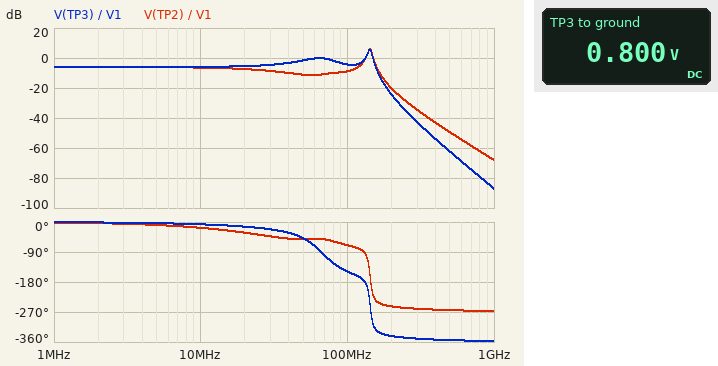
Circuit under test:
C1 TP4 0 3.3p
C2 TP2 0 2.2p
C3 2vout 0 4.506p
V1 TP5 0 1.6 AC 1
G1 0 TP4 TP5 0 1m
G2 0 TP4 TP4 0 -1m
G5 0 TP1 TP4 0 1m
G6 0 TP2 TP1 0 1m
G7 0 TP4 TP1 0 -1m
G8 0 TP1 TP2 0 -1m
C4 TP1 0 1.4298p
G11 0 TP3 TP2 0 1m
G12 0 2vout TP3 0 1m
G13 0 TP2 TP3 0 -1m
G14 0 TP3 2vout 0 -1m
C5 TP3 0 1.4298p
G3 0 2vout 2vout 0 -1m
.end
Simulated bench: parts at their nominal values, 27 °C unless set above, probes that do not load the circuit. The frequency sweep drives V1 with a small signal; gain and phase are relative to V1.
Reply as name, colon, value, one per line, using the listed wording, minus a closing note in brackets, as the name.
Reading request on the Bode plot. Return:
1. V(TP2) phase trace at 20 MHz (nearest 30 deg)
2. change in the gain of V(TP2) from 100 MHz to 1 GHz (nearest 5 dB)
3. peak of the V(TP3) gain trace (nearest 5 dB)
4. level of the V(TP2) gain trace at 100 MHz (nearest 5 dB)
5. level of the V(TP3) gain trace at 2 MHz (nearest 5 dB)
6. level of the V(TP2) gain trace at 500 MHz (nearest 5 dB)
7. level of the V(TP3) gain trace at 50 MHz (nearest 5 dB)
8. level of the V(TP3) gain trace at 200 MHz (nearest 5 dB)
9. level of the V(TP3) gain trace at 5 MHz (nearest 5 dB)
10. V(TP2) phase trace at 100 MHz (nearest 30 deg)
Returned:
V(TP2) phase trace at 20 MHz: -30 deg
change in the gain of V(TP2) from 100 MHz to 1 GHz: -60 dB
peak of the V(TP3) gain trace: 5 dB
level of the V(TP2) gain trace at 100 MHz: -10 dB
level of the V(TP3) gain trace at 2 MHz: -5 dB
level of the V(TP2) gain trace at 500 MHz: -50 dB
level of the V(TP3) gain trace at 50 MHz: 0 dB
level of the V(TP3) gain trace at 200 MHz: -25 dB
level of the V(TP3) gain trace at 5 MHz: -5 dB
V(TP2) phase trace at 100 MHz: -60 deg
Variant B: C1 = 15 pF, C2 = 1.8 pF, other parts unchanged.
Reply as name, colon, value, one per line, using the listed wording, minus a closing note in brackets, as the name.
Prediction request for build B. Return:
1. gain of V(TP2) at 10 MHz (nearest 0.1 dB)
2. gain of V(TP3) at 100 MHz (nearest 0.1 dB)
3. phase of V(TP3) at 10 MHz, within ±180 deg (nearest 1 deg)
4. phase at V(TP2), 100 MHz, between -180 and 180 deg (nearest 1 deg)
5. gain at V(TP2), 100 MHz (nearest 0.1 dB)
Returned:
gain of V(TP2) at 10 MHz: -7.4 dB
gain of V(TP3) at 100 MHz: -18.2 dB
phase of V(TP3) at 10 MHz, within ±180 deg: -24 deg
phase at V(TP2), 100 MHz, between -180 and 180 deg: -94 deg
gain at V(TP2), 100 MHz: -22.7 dB
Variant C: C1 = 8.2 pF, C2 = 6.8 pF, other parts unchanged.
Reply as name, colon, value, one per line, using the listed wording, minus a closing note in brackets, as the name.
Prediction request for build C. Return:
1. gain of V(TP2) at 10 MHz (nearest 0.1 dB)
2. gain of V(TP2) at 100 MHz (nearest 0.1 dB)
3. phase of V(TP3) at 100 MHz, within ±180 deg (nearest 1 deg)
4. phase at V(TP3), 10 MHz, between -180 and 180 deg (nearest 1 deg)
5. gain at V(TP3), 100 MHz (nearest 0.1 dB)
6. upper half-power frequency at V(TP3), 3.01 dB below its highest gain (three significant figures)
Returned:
gain of V(TP2) at 10 MHz: -7.2 dB
gain of V(TP2) at 100 MHz: -13.6 dB
phase of V(TP3) at 100 MHz, within ±180 deg: 42 deg
phase at V(TP3), 10 MHz, between -180 and 180 deg: -21 deg
gain at V(TP3), 100 MHz: -9.1 dB
upper half-power frequency at V(TP3), 3.01 dB below its highest gain: 93.7 MHz
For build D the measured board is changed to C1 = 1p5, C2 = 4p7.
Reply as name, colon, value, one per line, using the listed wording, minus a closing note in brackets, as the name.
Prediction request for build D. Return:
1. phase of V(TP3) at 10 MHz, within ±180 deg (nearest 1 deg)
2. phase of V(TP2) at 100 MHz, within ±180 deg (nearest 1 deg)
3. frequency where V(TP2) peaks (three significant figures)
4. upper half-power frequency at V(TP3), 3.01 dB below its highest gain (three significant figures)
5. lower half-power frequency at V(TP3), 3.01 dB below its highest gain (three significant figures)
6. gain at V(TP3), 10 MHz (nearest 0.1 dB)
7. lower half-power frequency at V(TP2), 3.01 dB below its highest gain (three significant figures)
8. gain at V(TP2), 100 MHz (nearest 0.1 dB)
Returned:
phase of V(TP3) at 10 MHz, within ±180 deg: -8 deg
phase of V(TP2) at 100 MHz, within ±180 deg: -95 deg
frequency where V(TP2) peaks: 105 MHz
upper half-power frequency at V(TP3), 3.01 dB below its highest gain: 114 MHz
lower half-power frequency at V(TP3), 3.01 dB below its highest gain: 60.2 MHz
gain at V(TP3), 10 MHz: -5.9 dB
lower half-power frequency at V(TP2), 3.01 dB below its highest gain: 82.5 MHz
gain at V(TP2), 100 MHz: -3.1 dB
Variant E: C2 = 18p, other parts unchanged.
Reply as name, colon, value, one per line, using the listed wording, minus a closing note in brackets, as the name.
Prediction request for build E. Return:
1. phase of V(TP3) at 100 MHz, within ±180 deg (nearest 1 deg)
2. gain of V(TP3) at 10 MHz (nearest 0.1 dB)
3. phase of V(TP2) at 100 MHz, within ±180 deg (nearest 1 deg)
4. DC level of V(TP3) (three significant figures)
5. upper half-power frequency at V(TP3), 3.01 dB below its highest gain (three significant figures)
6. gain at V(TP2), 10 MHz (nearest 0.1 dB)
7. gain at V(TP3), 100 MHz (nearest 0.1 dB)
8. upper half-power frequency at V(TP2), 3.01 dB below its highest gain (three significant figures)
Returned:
phase of V(TP3) at 100 MHz, within ±180 deg: 64 deg
gain of V(TP3) at 10 MHz: -7.4 dB
phase of V(TP2) at 100 MHz, within ±180 deg: 143 deg
DC level of V(TP3): 800 mV
upper half-power frequency at V(TP3), 3.01 dB below its highest gain: 81.1 MHz
gain at V(TP2), 10 MHz: -7.9 dB
gain at V(TP3), 100 MHz: -15.4 dB
upper half-power frequency at V(TP2), 3.01 dB below its highest gain: 13.6 MHz
